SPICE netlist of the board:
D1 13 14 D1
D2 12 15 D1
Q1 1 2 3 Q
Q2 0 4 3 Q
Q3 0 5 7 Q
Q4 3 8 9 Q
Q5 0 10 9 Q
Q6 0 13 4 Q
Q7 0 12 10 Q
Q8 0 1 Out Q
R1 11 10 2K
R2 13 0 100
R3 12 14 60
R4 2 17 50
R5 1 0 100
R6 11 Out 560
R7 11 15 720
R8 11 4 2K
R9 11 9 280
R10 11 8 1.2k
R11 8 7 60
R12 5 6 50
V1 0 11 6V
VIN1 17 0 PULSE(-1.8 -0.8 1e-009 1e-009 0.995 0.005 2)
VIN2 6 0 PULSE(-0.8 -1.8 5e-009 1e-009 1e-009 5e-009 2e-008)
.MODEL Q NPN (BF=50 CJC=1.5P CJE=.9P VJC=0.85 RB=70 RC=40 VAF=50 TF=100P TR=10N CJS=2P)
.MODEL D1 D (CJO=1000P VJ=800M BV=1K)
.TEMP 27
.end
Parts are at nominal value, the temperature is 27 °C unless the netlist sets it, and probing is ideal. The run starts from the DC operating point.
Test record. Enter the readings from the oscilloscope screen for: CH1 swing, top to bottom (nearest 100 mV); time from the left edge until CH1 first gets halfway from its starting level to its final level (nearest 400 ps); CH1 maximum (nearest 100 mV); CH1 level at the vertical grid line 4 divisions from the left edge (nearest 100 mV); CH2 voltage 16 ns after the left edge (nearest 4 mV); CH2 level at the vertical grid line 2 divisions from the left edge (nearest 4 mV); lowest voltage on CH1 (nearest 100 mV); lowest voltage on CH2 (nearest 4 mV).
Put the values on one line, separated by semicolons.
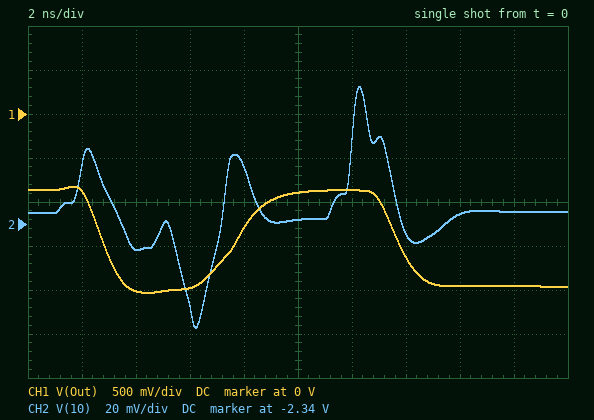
1.2 V; 2.8 ns; -800 mV; -1.3 V; -2.336 V; -2.352 V; -2.0 V; -2.388 V
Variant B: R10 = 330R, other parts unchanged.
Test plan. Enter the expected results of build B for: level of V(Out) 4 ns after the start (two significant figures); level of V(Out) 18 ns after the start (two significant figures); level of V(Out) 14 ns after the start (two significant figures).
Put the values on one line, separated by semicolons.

-1.5 V; -1.3 V; -870 mV
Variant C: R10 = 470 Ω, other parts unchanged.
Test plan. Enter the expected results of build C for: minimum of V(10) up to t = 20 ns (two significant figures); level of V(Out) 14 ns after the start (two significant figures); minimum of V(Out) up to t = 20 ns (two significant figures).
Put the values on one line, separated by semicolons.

-2.4 V; -1.1 V; -1.9 V
